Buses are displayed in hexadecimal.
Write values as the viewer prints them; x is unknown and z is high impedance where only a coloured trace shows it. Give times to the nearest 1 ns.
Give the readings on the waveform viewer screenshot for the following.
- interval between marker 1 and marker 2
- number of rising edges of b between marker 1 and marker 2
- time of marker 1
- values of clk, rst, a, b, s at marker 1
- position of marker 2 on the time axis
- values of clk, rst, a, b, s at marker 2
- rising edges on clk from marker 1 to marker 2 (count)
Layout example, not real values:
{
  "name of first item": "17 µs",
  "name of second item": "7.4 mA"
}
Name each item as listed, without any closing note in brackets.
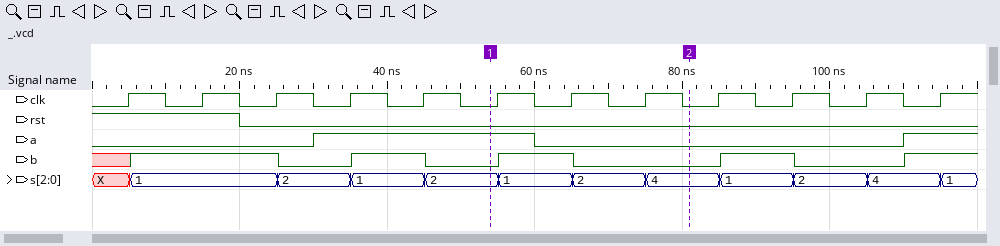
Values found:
{
  "interval between marker 1 and marker 2": "27 ns",
  "number of rising edges of b between marker 1 and marker 2": "1",
  "time of marker 1": "54 ns",
  "values of clk, rst, a, b, s at marker 1": "clk=0, rst=0, a=1, b=0, s=2",
  "position of marker 2 on the time axis": "81 ns",
  "values of clk, rst, a, b, s at marker 2": "clk=0, rst=0, a=0, b=0, s=4",
  "rising edges on clk from marker 1 to marker 2": "3"
}
